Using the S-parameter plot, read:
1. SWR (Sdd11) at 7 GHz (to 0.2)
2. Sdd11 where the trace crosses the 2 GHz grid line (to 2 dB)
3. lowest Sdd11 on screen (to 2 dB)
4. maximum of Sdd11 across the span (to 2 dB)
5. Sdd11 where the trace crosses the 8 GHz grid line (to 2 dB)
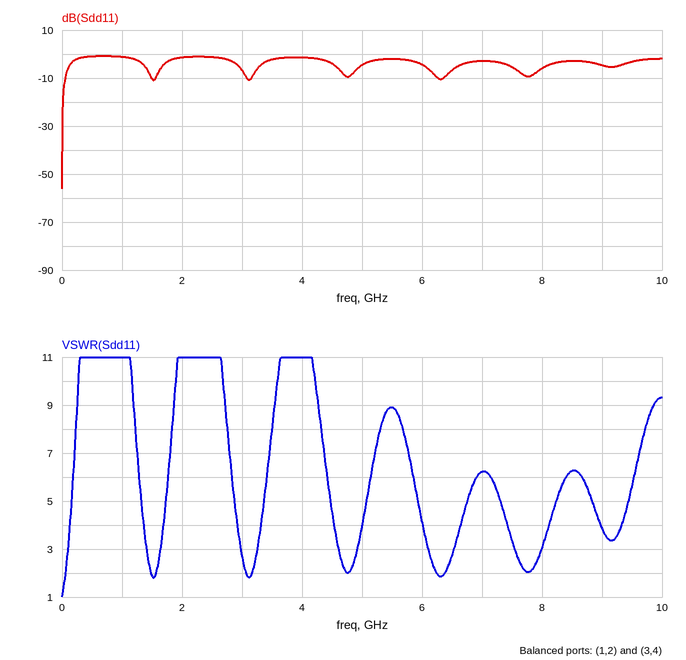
6.2
-2 dB
-56 dB
0 dB
-6 dB
